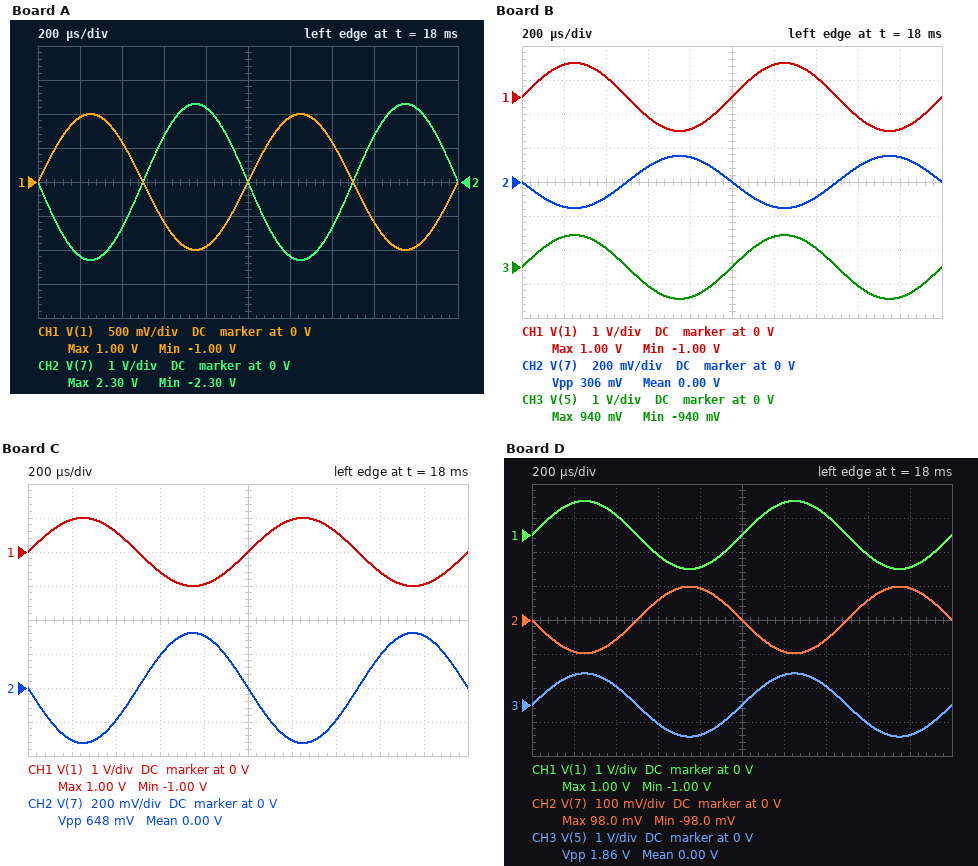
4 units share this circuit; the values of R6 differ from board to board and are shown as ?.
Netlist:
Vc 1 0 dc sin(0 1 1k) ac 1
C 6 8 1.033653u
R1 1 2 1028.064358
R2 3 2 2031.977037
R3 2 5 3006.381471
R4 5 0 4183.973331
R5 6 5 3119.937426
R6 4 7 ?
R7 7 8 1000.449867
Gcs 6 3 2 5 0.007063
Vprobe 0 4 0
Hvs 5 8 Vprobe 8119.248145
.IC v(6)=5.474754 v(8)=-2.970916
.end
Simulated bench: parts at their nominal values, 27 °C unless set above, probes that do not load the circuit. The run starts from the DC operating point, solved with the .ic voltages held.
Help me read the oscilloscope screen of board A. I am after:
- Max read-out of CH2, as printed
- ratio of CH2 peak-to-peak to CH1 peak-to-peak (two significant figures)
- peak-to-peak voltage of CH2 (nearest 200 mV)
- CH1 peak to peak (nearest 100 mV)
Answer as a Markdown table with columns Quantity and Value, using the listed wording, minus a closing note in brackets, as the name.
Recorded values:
| Quantity | Value |
|---|---|
| Max read-out of CH2, as printed | 2.30 V |
| ratio of CH2 peak-to-peak to CH1 peak-to-peak | 2.3 |
| peak-to-peak voltage of CH2 | 4.6 V |
| CH1 peak to peak | 2.0 V |
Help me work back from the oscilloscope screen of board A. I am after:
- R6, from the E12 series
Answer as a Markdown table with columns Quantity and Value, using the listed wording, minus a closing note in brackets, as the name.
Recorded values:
| Quantity | Value |
|---|---|
| R6, from the E12 series | 4.7 kΩ |
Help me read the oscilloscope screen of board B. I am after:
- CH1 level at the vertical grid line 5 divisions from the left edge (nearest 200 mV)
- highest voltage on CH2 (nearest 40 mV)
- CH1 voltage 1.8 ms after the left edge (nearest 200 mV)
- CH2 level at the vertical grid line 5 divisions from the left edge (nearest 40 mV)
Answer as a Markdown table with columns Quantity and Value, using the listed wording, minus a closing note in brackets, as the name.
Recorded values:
| Quantity | Value |
|---|---|
| CH1 level at the vertical grid line 5 divisions from the left edge | 0 V |
| highest voltage on CH2 | 160 mV |
| CH1 voltage 1.8 ms after the left edge | -1.0 V |
| CH2 level at the vertical grid line 5 divisions from the left edge | 0 V |
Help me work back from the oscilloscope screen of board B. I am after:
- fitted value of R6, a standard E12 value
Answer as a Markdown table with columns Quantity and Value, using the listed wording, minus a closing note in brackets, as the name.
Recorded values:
| Quantity | Value |
|---|---|
| fitted value of R6, a standard E12 value | 1 kΩ |
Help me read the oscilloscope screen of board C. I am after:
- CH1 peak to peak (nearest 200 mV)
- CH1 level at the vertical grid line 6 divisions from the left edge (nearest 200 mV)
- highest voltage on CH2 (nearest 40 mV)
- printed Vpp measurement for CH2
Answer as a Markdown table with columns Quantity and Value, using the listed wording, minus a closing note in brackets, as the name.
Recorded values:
| Quantity | Value |
|---|---|
| CH1 peak to peak | 2.0 V |
| CH1 level at the vertical grid line 6 divisions from the left edge | 1.0 V |
| highest voltage on CH2 | 320 mV |
| printed Vpp measurement for CH2 | 648 mV |
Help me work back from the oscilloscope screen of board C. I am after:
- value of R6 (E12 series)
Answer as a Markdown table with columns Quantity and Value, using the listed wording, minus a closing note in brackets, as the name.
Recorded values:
| Quantity | Value |
|---|---|
| value of R6 | 1.8 kΩ |
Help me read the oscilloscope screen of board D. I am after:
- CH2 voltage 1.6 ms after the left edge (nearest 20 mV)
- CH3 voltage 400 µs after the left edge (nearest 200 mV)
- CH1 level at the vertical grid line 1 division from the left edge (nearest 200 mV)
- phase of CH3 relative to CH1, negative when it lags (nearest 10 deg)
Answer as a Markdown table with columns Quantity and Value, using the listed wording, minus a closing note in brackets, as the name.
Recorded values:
| Quantity | Value |
|---|---|
| CH2 voltage 1.6 ms after the left edge | 60 mV |
| CH3 voltage 400 µs after the left edge | 600 mV |
| CH1 level at the vertical grid line 1 division from the left edge | 1.0 V |
| phase of CH3 relative to CH1, negative when it lags | 0 deg |
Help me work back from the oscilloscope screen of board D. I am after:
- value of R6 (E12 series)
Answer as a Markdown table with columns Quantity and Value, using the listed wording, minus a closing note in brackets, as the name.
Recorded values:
| Quantity | Value |
|---|---|
| value of R6 | 680 Ω |
